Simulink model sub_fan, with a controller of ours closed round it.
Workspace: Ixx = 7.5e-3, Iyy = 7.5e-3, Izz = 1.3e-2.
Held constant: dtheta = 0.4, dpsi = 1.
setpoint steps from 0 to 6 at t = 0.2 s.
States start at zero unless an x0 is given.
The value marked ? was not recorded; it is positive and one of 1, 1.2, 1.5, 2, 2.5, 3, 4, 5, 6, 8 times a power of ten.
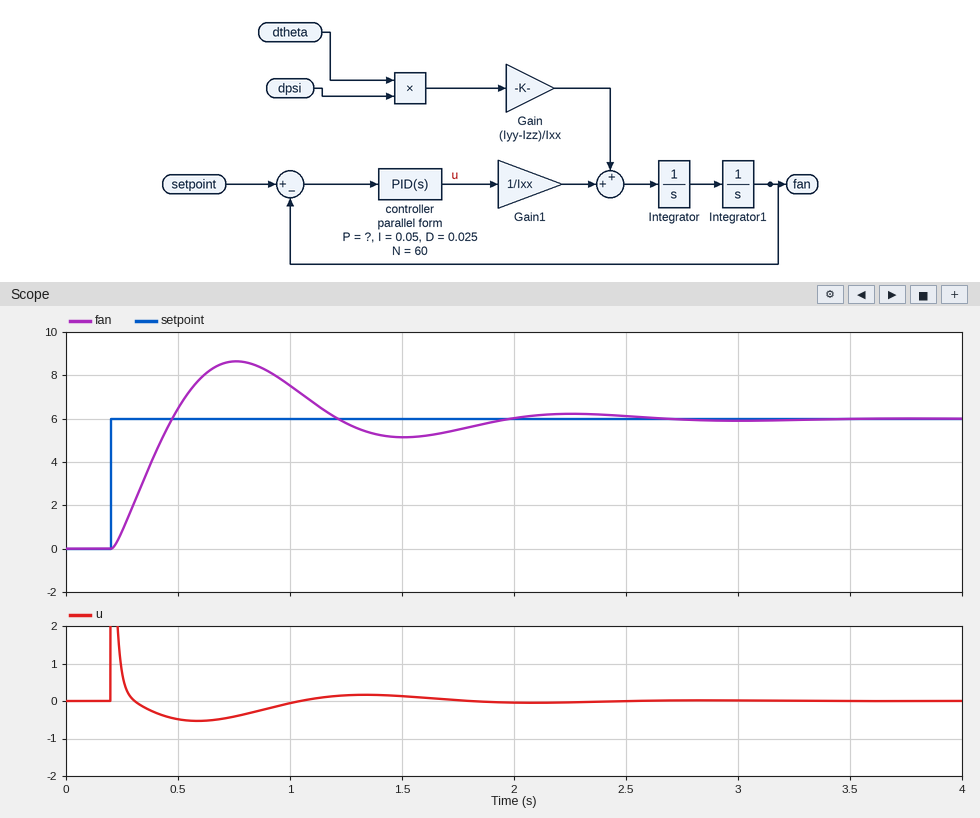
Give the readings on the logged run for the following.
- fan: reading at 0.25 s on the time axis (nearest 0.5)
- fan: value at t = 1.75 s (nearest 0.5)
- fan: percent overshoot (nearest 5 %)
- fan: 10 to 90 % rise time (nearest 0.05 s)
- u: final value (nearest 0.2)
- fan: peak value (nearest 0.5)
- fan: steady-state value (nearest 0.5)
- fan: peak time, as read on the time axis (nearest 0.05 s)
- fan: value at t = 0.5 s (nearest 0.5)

1.0
5.5
45 %
0.20 s
0.0
8.5
6.0
0.75 s
6.5
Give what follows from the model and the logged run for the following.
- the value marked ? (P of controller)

0.15
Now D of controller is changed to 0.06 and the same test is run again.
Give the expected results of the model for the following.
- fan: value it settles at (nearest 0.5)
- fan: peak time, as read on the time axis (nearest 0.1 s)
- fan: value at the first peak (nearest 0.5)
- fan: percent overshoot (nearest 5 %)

6.0
0.6 s
7.0
20 %
